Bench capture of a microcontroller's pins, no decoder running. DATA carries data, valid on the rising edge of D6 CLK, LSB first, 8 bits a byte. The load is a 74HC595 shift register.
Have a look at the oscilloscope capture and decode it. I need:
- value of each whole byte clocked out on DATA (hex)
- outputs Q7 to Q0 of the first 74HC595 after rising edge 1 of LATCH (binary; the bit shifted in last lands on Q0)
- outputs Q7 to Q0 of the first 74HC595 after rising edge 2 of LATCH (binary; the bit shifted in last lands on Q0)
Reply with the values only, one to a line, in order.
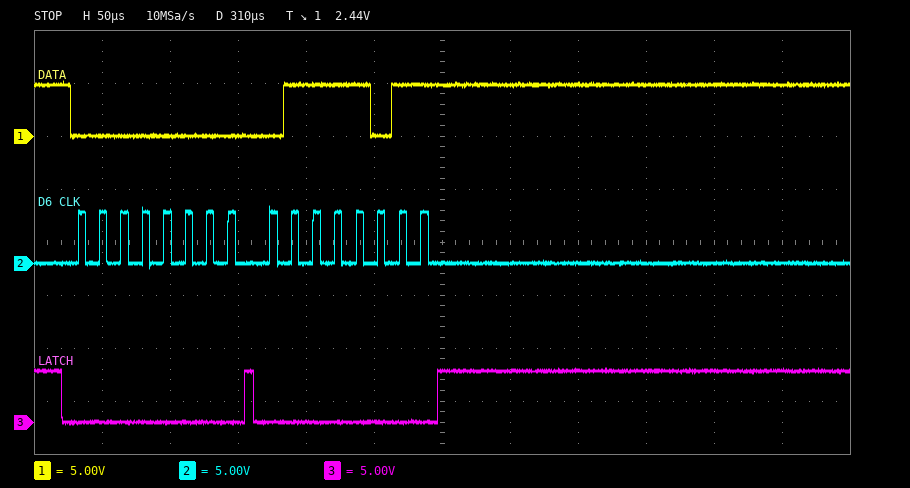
0x00 0xDE
00000000
01111011
